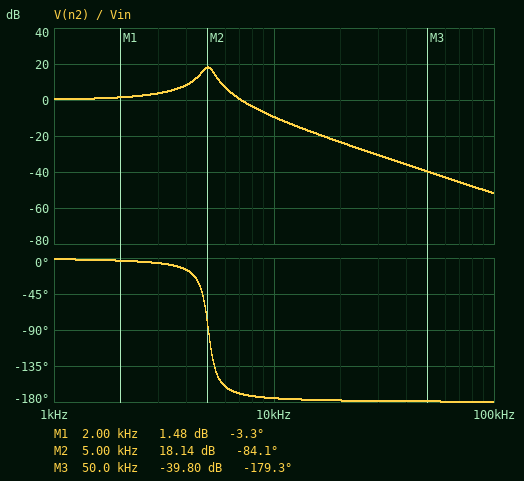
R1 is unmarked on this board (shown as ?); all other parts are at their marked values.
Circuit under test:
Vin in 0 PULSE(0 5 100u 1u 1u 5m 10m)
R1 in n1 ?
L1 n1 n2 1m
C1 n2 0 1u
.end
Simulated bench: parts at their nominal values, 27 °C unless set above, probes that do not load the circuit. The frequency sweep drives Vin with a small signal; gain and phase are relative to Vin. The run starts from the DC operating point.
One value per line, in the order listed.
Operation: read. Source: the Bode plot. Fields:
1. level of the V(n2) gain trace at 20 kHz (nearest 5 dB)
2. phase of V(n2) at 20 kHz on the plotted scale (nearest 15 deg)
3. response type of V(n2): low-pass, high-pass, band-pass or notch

-25 dB
-180 deg
low-pass
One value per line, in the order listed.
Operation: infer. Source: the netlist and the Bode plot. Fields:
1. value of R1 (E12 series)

3.9 Ω
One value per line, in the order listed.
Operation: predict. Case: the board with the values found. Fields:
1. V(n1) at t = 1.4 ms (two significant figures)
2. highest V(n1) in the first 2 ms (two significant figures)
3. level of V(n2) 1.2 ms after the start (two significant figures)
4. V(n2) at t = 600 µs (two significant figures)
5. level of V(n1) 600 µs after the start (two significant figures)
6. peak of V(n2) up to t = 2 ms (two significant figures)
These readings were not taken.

5.0 V
5.5 V
5.6 V
6.9 V
5.0 V
9.1 V
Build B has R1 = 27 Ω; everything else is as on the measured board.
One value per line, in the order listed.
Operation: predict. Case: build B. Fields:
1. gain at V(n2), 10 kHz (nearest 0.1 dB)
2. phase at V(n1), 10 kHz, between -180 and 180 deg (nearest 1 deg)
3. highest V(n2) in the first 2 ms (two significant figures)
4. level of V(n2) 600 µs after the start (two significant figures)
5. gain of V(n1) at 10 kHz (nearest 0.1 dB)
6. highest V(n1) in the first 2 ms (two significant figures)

-10.6 dB
30 deg
6.1 V
5.0 V
-1.2 dB
5.6 V
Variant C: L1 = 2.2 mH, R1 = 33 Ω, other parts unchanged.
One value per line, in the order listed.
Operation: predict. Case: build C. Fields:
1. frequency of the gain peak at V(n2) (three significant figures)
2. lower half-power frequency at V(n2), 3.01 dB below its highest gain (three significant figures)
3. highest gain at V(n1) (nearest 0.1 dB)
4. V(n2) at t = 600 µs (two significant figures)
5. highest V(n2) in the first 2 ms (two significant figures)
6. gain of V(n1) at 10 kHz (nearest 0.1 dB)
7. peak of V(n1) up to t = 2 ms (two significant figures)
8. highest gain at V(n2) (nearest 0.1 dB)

2.94 kHz
1.04 kHz
0 dB
5.1 V
6.5 V
-0.3 dB
5.7 V
3.6 dB
